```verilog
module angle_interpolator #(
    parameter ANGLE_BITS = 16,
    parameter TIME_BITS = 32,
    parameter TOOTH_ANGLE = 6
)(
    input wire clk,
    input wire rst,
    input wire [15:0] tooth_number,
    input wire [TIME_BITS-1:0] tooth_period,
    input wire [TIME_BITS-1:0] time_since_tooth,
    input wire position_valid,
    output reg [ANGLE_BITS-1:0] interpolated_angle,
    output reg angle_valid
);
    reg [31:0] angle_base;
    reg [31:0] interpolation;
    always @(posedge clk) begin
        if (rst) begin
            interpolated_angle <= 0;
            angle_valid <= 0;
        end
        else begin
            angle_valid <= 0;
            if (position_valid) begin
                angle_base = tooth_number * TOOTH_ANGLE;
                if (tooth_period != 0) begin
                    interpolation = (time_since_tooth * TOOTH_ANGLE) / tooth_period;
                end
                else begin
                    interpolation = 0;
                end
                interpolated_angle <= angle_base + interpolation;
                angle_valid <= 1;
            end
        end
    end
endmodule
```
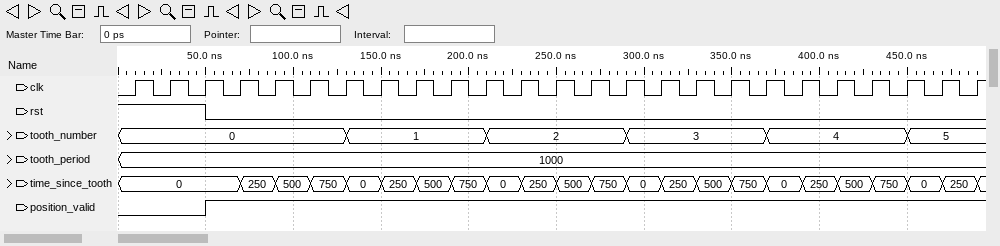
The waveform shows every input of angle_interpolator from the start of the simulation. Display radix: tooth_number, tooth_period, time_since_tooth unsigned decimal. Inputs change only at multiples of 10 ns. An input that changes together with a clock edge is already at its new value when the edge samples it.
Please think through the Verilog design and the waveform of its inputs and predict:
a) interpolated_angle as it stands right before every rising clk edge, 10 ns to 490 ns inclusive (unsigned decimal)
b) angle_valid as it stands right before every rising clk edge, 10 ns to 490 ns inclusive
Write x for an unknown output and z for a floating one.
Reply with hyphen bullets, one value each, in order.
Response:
- x, 0, 0, 0, 1, 3, 4, 6, 7, 9, 10, 12, 13, 15, 16, 18, 19, 21, 22, 24, 25, 27, 28, 30, 31
- x 0 0 1 1 1 1 1 1 1 1 1 1 1 1 1 1 1 1 1 1 1 1 1 1
